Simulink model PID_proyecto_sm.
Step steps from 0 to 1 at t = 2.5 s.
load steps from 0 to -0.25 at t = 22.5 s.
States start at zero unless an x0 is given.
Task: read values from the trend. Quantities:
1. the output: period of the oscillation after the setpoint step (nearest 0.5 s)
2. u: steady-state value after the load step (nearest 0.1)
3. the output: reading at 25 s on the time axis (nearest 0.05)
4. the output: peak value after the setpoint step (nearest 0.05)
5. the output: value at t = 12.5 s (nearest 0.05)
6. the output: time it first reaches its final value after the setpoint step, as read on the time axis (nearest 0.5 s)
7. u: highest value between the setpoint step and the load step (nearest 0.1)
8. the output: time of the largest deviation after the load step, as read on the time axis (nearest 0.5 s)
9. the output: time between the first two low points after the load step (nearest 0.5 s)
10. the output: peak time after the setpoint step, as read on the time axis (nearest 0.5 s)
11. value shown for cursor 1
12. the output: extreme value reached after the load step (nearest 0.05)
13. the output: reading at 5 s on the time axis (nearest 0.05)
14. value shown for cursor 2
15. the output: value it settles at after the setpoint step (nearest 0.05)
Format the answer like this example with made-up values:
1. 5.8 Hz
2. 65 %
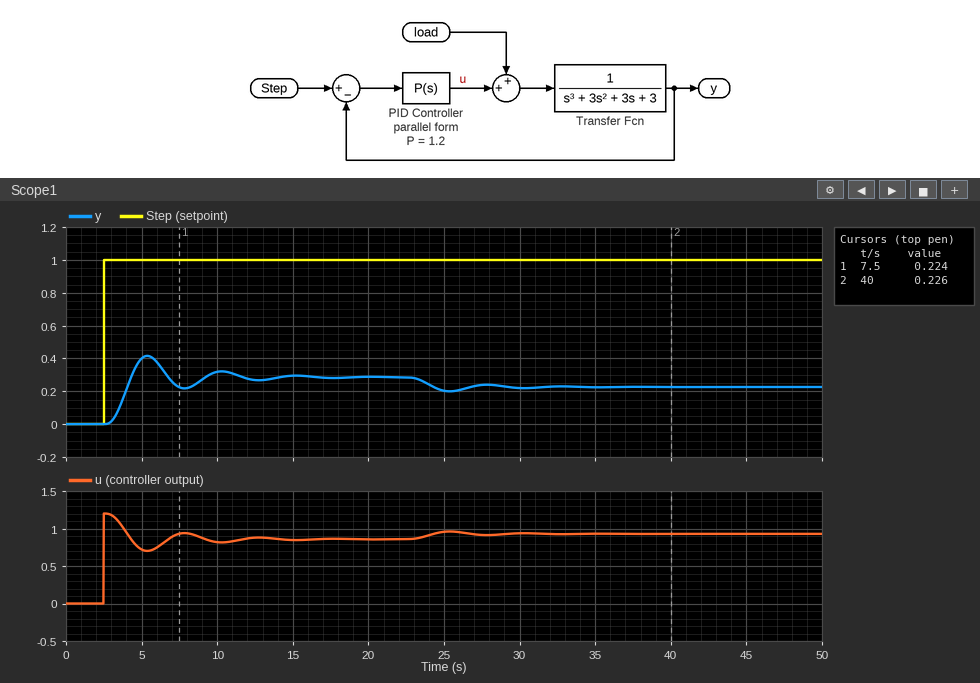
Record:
1. 5.0 s
2. 0.9
3. 0.20
4. 0.40
5. 0.25
6. 4.5 s
7. 1.2
8. 25.5 s
9. 5.0 s
10. 5.5 s
11. 0.224
12. 0.20
13. 0.40
14. 0.226
15. 0.30
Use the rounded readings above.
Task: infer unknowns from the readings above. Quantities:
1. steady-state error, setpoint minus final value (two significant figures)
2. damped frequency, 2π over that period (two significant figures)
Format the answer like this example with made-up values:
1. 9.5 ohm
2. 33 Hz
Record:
1. 0.70
2. 1.3 rad/s
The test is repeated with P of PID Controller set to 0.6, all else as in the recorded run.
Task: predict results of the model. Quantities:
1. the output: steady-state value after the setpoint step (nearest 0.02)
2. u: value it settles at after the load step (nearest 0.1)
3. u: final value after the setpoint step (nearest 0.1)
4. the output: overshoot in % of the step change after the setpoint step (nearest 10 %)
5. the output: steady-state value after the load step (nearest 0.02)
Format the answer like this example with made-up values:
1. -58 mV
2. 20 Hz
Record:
1. 0.16
2. 0.5
3. 0.5
4. 40 %
5. 0.10
